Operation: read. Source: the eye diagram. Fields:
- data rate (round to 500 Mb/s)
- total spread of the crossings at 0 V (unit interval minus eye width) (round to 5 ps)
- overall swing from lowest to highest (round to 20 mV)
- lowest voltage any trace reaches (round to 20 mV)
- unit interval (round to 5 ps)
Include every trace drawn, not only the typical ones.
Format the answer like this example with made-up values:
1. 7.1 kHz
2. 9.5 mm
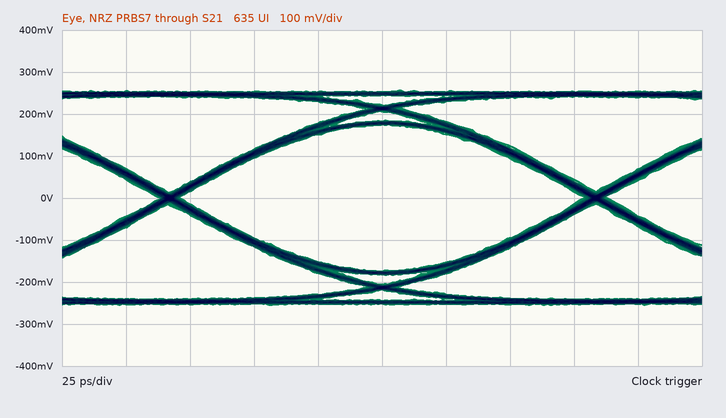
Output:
1. 6.0 Gb/s
2. 10 ps
3. 520 mV
4. -260 mV
5. 165 ps
